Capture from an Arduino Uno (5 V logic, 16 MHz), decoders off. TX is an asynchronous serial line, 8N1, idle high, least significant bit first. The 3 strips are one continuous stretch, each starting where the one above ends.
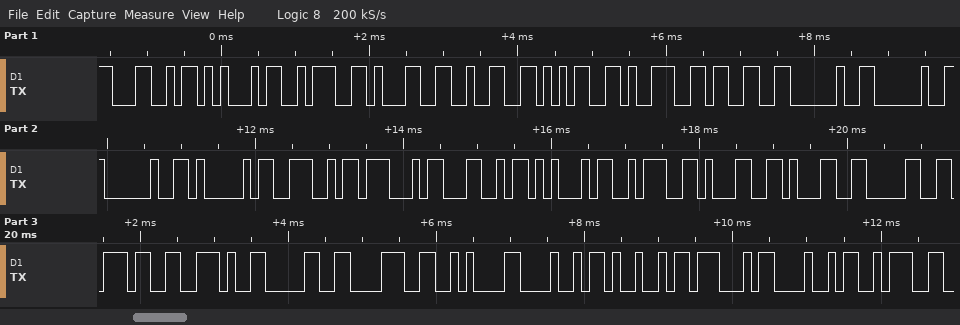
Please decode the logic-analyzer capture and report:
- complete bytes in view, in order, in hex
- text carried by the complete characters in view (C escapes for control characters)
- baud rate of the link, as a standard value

4C 45 3A 31 32 35 39 33 20 20 20 41 4E 47 4C 45 3A 31 31 30 37 2E 30 38 0A 48 49 47 48 3A
"LE:12593   ANGLE:1107.08\nHIGH:"
9600 baud
